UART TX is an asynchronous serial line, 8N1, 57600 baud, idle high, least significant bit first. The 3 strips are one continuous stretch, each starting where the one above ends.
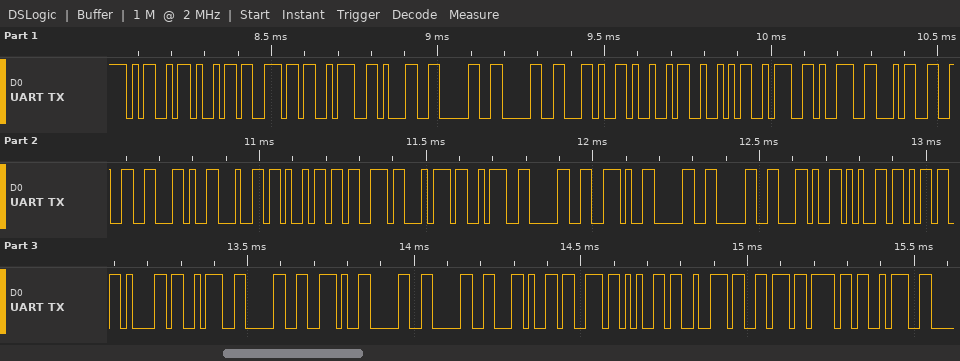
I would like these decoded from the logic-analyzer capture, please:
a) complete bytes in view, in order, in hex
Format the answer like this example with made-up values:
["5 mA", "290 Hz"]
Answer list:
["4D 69 6E 3A 31 30 30 2C 49 52 3A 39 34 32 2C 64 69 73 74 3A 30 2E 30 30 2C 65 6D 61 3A 30 2E 30 30 2C 73 65 72 76 6F 3A"]
